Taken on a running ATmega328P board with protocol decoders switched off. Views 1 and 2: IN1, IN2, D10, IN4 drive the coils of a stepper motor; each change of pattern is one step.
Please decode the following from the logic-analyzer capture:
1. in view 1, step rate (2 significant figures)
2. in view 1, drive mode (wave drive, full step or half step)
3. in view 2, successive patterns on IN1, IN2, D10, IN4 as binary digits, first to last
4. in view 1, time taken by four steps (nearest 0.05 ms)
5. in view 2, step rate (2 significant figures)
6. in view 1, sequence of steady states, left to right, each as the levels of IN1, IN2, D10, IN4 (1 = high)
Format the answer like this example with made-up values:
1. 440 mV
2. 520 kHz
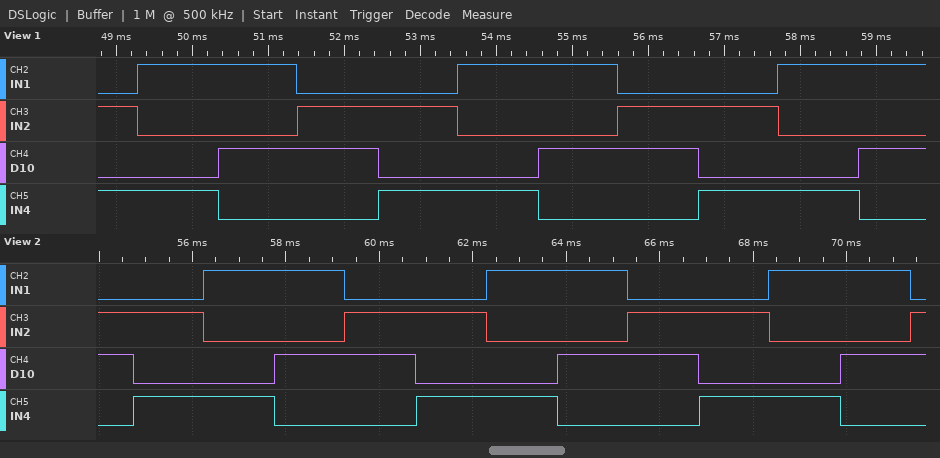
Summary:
1. 950 steps/s
2. full step
3. 0110 0101 1001 1010 0110 0101 1001 1010 0110 0101 1001 1010 0110
4. 4.20 ms
5. 660 steps/s
6. 0101 1001 1010 0110 0101 1001 1010 0110 0101 1001 1010
